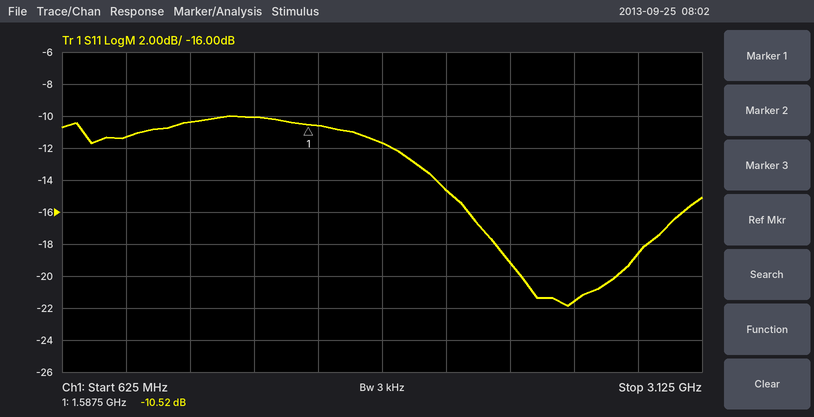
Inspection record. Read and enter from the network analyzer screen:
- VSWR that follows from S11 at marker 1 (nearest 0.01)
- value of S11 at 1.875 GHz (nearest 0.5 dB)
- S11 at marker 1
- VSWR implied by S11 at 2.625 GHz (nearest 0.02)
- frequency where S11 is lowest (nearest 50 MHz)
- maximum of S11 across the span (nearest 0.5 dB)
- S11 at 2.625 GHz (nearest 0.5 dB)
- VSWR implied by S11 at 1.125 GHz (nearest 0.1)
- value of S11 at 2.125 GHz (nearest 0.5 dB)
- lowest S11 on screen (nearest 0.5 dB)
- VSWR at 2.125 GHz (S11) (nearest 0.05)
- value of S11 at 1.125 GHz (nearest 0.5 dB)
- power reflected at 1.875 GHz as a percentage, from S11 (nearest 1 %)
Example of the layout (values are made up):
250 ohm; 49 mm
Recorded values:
1.85; -11.5 dB; -10.52 dB; 1.18; 2.60 GHz; -10.0 dB; -21.5 dB; 1.9; -14.5 dB; -22.0 dB; 1.45; -10.5 dB; 7 %
